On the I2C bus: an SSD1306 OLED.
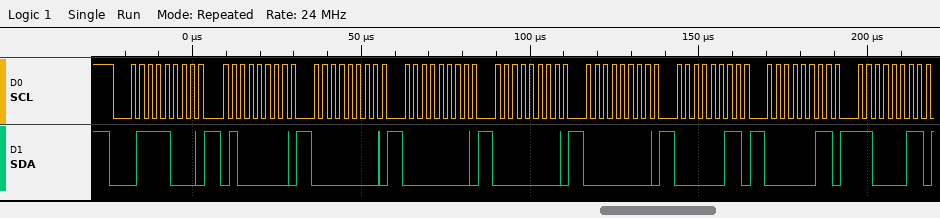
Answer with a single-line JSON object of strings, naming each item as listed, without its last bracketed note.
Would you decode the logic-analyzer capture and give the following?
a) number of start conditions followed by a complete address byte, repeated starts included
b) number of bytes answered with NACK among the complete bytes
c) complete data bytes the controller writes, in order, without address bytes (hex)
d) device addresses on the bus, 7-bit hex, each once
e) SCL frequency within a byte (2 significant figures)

{"number of start conditions followed by a complete address byte, repeated starts included": "1", "number of bytes answered with NACK among the complete bytes": "0", "complete data bytes the controller writes, in order, without address bytes": "40 00 00 00 00 03 03 C3", "device addresses on the bus, 7-bit hex, each once": "0x3C", "SCL frequency within a byte": "400 kHz"}
